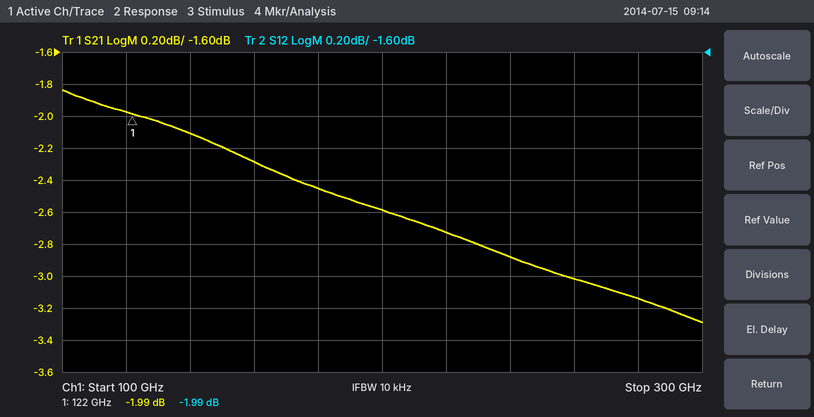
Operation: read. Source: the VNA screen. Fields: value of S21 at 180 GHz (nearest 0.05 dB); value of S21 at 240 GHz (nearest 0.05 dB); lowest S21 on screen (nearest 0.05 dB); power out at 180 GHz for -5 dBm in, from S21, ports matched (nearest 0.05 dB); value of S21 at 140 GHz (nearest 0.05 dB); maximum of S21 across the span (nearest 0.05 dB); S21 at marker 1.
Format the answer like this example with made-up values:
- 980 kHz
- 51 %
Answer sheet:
- -2.45 dB
- -2.90 dB
- -3.30 dB
- -7.45 dBm
- -2.10 dB
- -1.85 dB
- -1.99 dB
